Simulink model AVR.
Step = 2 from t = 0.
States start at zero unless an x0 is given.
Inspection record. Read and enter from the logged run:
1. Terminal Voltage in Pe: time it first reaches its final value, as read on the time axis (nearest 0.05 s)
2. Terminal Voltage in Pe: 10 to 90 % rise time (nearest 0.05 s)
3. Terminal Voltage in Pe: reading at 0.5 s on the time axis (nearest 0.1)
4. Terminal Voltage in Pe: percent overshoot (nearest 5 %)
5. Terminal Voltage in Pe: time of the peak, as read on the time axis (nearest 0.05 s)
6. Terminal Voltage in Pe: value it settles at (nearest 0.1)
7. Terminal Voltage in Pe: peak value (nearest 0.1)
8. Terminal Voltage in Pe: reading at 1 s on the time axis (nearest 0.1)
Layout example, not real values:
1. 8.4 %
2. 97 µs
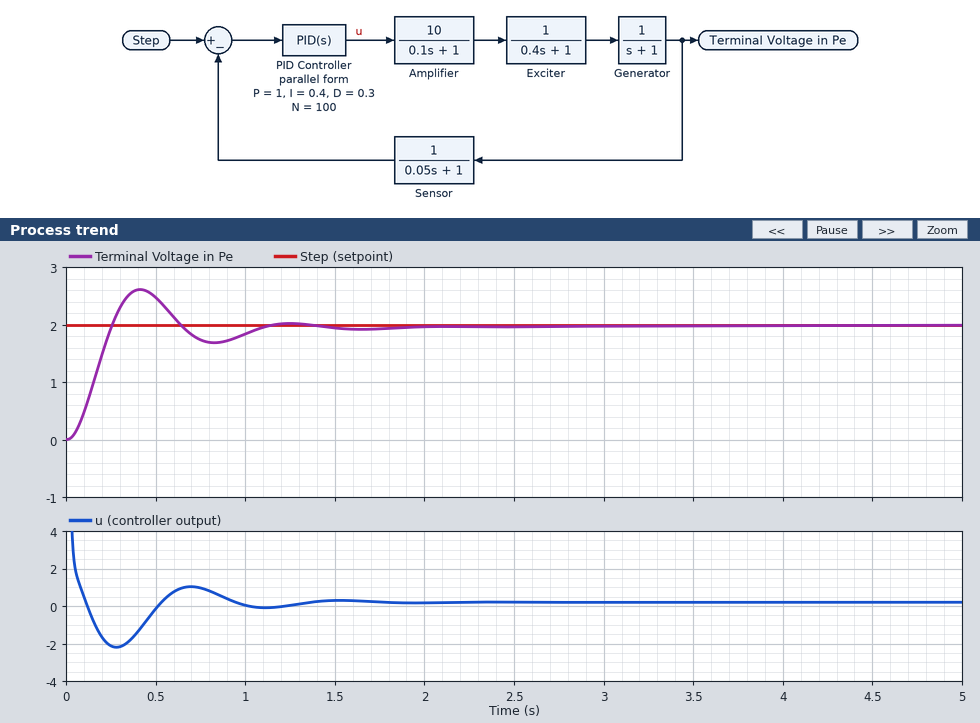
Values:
1. 0.25 s
2. 0.15 s
3. 2.5
4. 30 %
5. 0.40 s
6. 2.0
7. 2.6
8. 1.8
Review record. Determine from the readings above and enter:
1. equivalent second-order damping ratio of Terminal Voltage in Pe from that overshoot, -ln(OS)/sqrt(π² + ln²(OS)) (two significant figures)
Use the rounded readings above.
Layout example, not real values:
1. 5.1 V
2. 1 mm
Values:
1. 0.36
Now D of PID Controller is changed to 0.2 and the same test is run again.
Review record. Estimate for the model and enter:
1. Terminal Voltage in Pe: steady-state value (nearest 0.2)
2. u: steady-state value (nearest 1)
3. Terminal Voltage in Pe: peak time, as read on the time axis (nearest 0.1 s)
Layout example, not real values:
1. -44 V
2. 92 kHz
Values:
1. 2.0
2. 0
3. 0.5 s
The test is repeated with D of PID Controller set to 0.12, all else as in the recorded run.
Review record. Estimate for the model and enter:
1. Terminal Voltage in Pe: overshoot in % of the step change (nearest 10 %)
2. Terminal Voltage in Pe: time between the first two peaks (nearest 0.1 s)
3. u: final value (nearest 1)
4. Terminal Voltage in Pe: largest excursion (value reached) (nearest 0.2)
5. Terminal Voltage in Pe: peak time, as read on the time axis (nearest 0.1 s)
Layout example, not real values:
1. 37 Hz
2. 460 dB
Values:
1. 40 %
2. 1.3 s
3. 0
4. 2.8
5. 0.6 s
